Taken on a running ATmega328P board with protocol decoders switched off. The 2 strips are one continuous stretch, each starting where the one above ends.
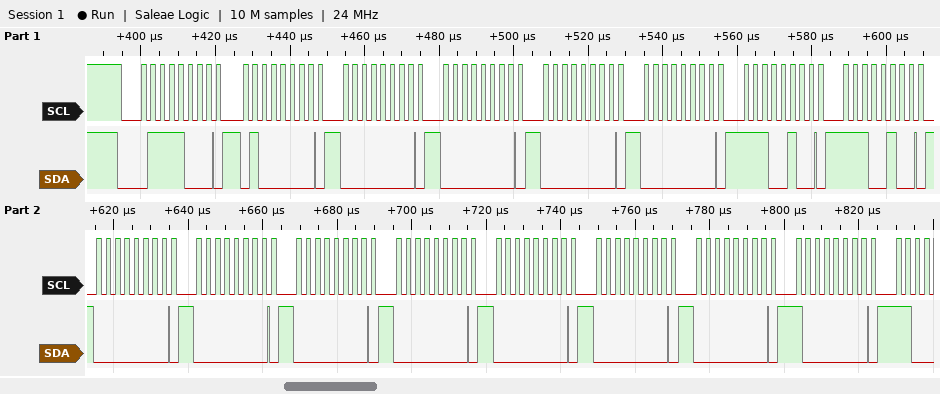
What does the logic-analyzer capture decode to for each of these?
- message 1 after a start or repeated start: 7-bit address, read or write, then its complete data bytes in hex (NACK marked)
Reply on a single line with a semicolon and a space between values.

0x3C write: 40 00 00 00 00 E4 E4 00 00 00 00 00 00 00 80
